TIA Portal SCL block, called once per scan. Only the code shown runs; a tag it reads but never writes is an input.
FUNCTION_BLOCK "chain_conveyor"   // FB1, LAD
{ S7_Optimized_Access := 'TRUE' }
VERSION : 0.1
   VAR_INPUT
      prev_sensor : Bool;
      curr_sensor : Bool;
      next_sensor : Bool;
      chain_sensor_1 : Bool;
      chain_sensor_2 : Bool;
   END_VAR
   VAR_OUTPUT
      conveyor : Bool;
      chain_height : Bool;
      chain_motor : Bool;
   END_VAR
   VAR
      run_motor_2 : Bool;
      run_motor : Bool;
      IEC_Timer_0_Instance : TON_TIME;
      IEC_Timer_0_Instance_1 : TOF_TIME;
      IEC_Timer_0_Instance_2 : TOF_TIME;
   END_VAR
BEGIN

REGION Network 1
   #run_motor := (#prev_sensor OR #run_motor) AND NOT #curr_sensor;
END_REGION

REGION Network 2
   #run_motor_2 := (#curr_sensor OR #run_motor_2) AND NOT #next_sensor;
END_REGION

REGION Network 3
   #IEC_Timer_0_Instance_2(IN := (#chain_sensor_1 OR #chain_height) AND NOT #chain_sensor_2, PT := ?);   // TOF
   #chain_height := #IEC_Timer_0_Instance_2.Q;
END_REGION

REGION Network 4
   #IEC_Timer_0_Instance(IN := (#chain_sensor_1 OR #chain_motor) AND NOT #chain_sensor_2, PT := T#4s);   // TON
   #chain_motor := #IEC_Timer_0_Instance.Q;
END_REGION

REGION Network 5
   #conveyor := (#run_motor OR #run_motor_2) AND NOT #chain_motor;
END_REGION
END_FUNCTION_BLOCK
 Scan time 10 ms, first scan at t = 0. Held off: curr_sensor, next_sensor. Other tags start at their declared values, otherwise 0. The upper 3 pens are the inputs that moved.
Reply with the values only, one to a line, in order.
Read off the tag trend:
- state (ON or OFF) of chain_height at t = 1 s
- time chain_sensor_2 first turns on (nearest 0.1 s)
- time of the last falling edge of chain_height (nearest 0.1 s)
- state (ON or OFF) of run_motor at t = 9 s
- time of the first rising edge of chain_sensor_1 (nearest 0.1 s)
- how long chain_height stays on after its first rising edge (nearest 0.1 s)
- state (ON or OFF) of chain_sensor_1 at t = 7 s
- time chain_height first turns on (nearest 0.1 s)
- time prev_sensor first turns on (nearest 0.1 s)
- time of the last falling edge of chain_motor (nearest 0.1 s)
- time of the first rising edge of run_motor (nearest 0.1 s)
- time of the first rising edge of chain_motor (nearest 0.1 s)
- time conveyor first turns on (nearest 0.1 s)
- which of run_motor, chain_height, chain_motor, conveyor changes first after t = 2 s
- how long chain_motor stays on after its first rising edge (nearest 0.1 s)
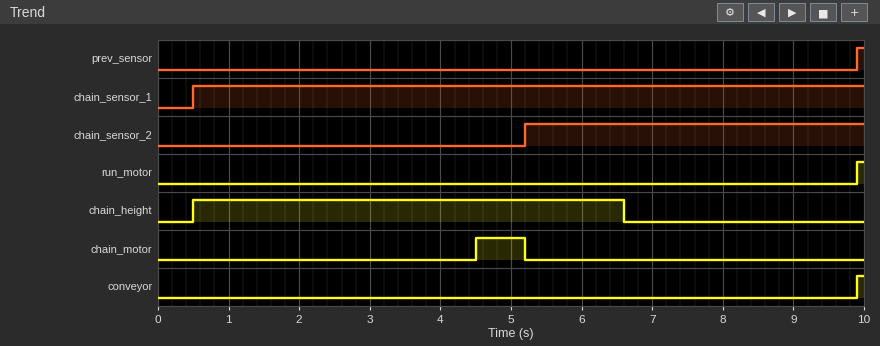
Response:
ON
5.2 s
6.6 s
OFF
0.5 s
6.1 s
ON
0.5 s
9.9 s
5.2 s
9.9 s
4.5 s
9.9 s
chain_motor
0.7 s
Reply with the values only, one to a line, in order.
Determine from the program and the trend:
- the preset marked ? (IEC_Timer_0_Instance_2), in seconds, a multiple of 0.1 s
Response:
1.4 s
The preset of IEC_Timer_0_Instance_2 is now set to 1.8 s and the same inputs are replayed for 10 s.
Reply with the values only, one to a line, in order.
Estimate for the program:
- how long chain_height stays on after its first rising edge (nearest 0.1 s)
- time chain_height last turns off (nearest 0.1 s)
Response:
6.5 s
7.0 s
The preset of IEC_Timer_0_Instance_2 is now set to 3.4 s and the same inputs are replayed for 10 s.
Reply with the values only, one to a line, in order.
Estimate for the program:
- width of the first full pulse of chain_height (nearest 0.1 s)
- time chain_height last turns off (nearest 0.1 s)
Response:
8.1 s
8.6 s
